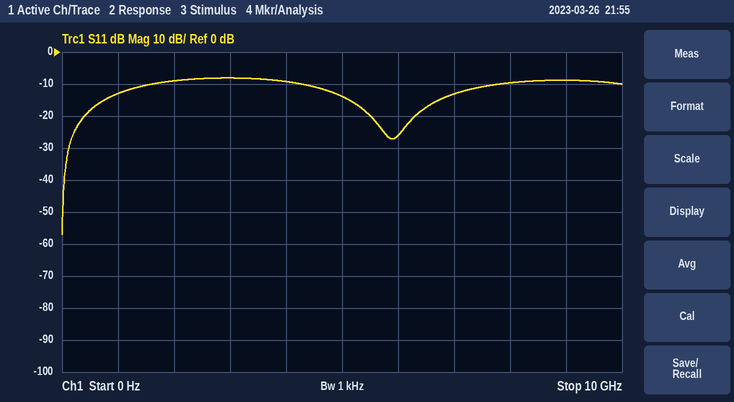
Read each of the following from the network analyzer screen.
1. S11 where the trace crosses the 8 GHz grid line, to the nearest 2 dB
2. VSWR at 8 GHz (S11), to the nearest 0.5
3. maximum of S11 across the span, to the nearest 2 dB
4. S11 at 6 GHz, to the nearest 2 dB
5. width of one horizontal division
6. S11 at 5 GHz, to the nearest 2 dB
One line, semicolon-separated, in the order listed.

-10 dB; 2.0; -8 dB; -26 dB; 1 GHz; -14 dB
